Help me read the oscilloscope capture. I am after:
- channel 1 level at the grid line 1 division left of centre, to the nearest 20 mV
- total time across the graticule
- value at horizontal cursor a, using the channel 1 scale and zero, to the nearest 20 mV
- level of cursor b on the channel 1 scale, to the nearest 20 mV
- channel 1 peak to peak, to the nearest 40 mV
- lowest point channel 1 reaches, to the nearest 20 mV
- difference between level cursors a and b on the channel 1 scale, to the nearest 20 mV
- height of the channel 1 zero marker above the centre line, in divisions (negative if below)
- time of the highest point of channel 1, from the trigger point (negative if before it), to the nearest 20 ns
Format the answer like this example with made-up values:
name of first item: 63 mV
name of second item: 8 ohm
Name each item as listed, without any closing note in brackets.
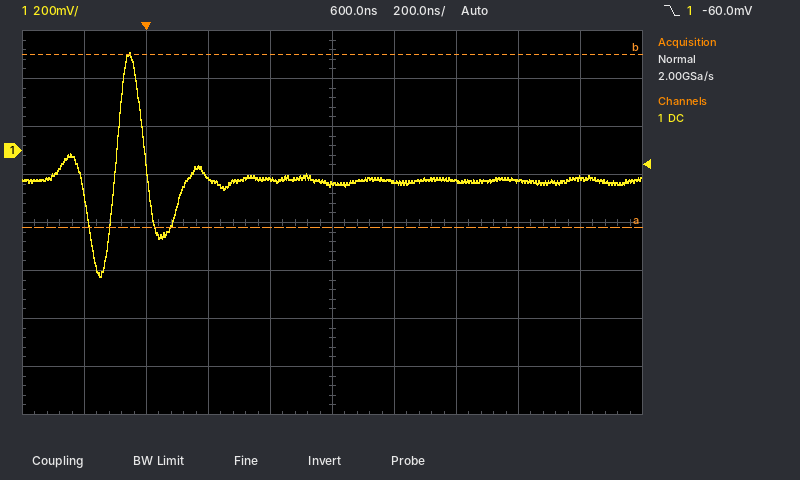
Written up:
channel 1 level at the grid line 1 division left of centre, to the nearest 20 mV: -120 mV
total time across the graticule: 2 µs
value at horizontal cursor a, using the channel 1 scale and zero, to the nearest 20 mV: -320 mV
level of cursor b on the channel 1 scale, to the nearest 20 mV: 400 mV
channel 1 peak to peak, to the nearest 40 mV: 920 mV
lowest point channel 1 reaches, to the nearest 20 mV: -520 mV
difference between level cursors a and b on the channel 1 scale, to the nearest 20 mV: 720 mV
height of the channel 1 zero marker above the centre line, in divisions: +1.5 div
time of the highest point of channel 1, from the trigger point (negative if before it), to the nearest 20 ns: -60 ns
